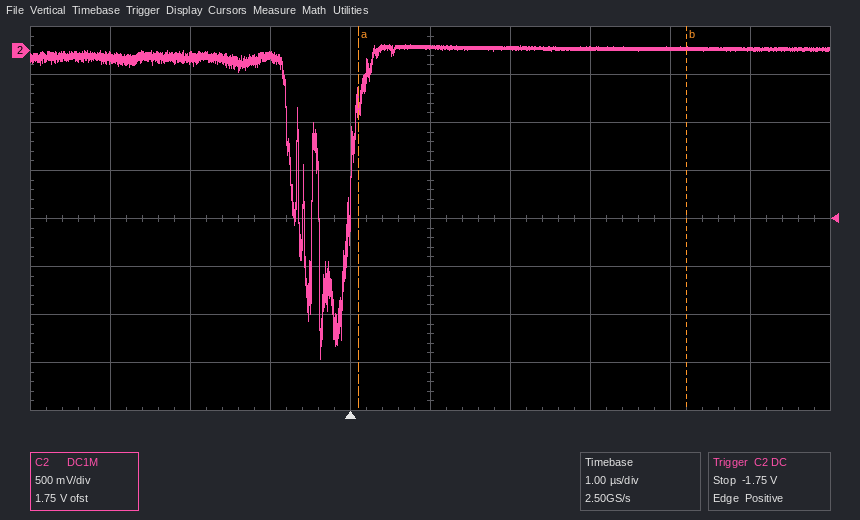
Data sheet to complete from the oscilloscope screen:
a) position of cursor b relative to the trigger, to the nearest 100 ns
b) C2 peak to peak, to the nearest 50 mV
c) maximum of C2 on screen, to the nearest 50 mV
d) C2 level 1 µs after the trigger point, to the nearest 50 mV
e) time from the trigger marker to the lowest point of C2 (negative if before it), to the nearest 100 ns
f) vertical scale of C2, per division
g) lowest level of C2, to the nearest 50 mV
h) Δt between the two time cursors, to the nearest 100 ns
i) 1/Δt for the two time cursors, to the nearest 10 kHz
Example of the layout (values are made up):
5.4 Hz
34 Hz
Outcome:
+4.2 µs
3.25 V
50 mV
50 mV
-400 ns
500 mV
-3.20 V
4.1 µs
240 kHz
